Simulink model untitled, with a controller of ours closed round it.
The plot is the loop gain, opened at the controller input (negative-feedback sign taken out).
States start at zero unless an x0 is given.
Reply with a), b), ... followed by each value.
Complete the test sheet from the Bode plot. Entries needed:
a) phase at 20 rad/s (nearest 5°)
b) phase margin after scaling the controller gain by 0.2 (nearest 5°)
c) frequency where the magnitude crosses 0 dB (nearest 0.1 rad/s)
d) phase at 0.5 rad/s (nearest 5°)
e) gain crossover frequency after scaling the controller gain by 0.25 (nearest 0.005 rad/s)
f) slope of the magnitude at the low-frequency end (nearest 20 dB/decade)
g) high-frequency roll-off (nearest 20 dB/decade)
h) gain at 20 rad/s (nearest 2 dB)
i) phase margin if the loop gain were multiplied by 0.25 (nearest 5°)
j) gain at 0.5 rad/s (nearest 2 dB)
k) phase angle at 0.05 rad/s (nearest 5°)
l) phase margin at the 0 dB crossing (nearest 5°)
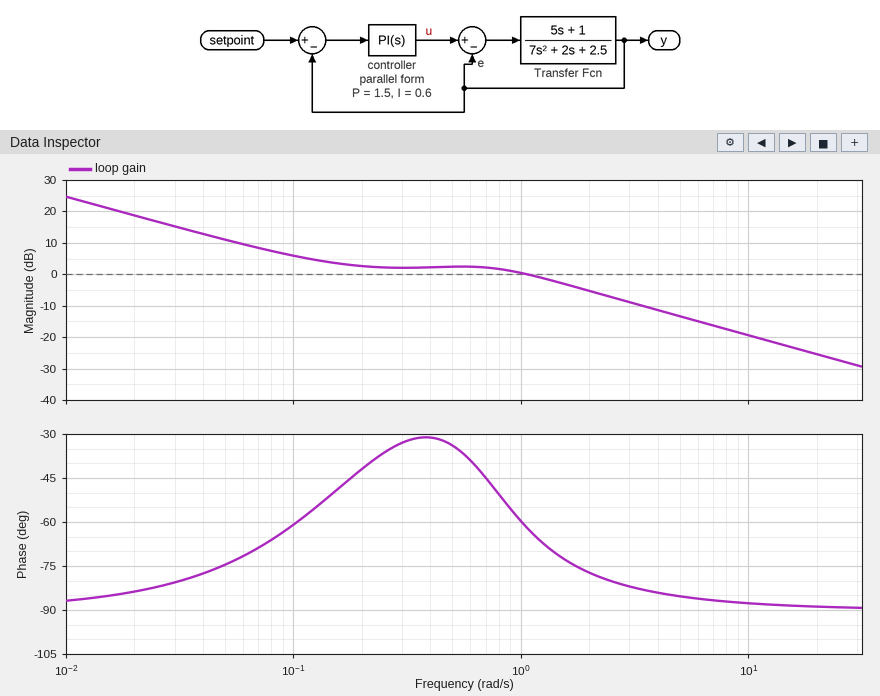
a) -90°
b) 100°
c) 1.1 rad/s
d) -35°
e) 0.045 rad/s
f) -20 dB/decade
g) -20 dB/decade
h) -26 dB
i) 105°
j) 2 dB
k) -75°
l) 120°
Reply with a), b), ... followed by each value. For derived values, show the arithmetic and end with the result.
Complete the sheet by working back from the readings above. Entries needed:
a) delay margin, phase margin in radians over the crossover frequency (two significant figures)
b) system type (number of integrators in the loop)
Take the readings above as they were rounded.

a) 120 × π / 180 / 1.1 = 1.9 s
b) 1
